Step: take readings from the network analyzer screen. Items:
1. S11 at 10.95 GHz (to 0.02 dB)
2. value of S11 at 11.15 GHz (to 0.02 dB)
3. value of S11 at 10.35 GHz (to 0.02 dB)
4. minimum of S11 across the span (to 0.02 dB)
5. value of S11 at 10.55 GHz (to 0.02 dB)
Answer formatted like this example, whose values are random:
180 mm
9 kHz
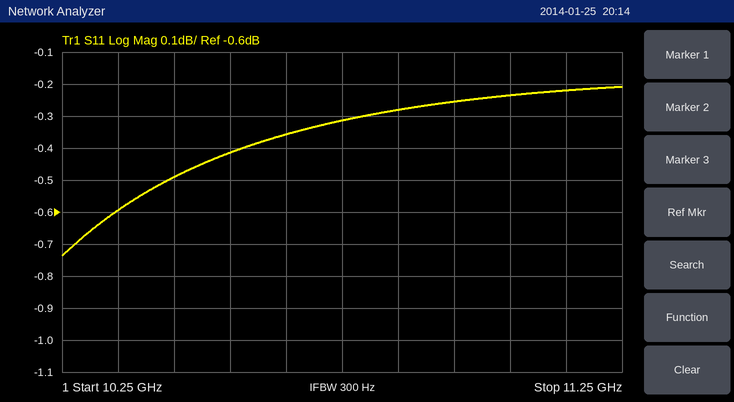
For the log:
-0.26 dB
-0.22 dB
-0.60 dB
-0.74 dB
-0.42 dB
